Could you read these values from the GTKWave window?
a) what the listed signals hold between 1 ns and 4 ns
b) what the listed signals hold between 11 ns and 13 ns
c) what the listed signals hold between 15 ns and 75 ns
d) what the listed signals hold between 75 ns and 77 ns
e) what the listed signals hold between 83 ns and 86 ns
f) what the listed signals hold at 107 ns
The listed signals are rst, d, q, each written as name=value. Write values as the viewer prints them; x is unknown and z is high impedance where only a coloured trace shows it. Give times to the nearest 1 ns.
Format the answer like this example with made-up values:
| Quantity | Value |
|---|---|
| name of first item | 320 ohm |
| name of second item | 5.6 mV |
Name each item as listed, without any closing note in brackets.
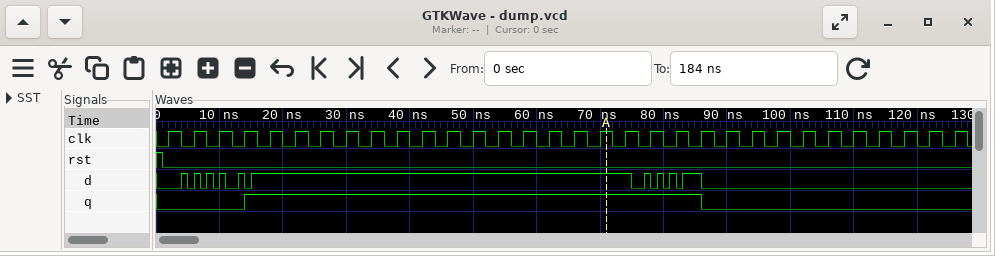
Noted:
| Quantity | Value |
|---|---|
| what the listed signals hold between 1 ns and 4 ns | rst=0, d=0, q=0 |
| what the listed signals hold between 11 ns and 13 ns | rst=0, d=0, q=0 |
| what the listed signals hold between 15 ns and 75 ns | rst=0, d=1, q=1 |
| what the listed signals hold between 75 ns and 77 ns | rst=0, d=0, q=1 |
| what the listed signals hold between 83 ns and 86 ns | rst=0, d=1, q=1 |
| what the listed signals hold at 107 ns | rst=0, d=0, q=0 |
